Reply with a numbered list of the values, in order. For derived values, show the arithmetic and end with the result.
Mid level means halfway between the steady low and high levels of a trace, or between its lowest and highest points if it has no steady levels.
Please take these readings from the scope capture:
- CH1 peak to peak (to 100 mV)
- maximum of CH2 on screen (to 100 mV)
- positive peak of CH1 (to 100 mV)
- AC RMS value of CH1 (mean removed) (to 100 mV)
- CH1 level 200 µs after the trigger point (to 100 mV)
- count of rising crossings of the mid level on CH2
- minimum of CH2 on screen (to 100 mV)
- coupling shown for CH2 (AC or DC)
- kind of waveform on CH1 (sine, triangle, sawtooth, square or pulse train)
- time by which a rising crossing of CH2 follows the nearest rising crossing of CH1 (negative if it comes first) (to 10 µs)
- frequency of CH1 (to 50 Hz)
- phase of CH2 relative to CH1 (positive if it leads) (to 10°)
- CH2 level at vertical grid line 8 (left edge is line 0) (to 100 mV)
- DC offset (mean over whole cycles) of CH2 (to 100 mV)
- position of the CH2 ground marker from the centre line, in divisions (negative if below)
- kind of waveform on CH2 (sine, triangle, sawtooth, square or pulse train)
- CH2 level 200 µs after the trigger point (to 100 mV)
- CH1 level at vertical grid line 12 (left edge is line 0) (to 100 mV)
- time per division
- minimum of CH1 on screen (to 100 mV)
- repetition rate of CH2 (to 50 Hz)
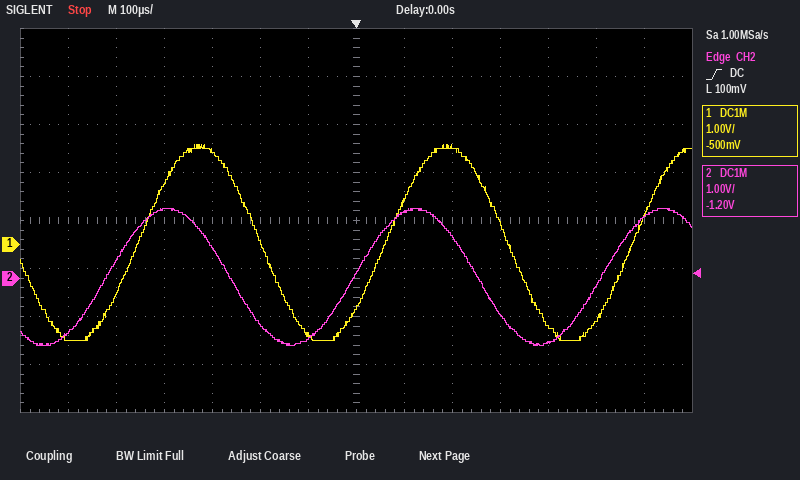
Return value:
1. 2.1 V − (-2.0 V) = 4.1 V
2. 1.4 V
3. 2.1 V
4. 4.1 V / (2√2) ≈ 1.4 V
5. 2.0 V
6. 3
7. -1.4 V
8. DC
9. sine
10. -70 µs
11. 1.95 kHz
12. +50°
13. 1.4 V
14. (1.4 V + (-1.4 V)) / 2 ≈ 0.0 V
15. -1.2 div
16. sine
17. 900 mV
18. -1.6 V
19. 100 µs
20. -2.0 V
21. 1.95 kHz
